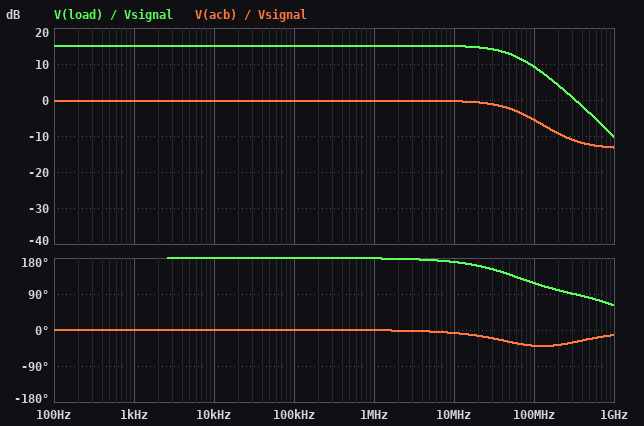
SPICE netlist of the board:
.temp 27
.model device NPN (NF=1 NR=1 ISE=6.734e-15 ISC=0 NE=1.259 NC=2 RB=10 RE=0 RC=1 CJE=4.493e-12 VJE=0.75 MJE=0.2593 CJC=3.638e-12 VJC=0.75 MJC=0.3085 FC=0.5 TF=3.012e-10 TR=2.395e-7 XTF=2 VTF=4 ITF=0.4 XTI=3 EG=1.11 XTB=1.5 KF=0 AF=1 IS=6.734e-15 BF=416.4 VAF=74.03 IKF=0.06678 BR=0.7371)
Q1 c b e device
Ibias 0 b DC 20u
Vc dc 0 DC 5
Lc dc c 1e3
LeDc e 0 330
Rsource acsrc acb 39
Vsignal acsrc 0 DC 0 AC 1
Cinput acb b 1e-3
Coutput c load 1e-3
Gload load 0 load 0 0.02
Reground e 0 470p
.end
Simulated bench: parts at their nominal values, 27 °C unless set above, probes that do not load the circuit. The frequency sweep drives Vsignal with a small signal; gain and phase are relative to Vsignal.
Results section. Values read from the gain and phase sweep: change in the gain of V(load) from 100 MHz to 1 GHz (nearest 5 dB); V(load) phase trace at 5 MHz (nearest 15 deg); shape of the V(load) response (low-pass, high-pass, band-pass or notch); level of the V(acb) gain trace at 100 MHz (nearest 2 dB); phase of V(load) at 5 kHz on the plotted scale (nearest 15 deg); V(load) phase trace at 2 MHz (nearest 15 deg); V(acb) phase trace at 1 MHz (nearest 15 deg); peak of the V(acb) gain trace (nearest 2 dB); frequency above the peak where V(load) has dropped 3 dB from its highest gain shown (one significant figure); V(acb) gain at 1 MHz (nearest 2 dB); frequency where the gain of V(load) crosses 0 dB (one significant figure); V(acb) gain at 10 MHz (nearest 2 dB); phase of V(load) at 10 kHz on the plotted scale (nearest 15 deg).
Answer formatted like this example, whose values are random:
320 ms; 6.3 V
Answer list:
-20 dB; 180 deg; low-pass; -6 dB; 180 deg; 180 deg; 0 deg; 0 dB; 60 MHz; 0 dB; 300 MHz; 0 dB; 180 deg
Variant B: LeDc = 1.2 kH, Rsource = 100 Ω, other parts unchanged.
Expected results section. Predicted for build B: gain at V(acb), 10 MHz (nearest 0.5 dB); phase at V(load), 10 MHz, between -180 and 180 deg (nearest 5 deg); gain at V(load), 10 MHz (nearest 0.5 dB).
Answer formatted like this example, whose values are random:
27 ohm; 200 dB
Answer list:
-1.0 dB; 160 deg; 14.0 dB
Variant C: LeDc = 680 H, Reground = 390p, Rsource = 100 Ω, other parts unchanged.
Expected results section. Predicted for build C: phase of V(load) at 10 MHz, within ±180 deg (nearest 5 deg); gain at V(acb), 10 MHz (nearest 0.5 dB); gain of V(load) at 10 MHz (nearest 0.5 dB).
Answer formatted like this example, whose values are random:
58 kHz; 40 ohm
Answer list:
160 deg; -1.0 dB; 14.0 dB
